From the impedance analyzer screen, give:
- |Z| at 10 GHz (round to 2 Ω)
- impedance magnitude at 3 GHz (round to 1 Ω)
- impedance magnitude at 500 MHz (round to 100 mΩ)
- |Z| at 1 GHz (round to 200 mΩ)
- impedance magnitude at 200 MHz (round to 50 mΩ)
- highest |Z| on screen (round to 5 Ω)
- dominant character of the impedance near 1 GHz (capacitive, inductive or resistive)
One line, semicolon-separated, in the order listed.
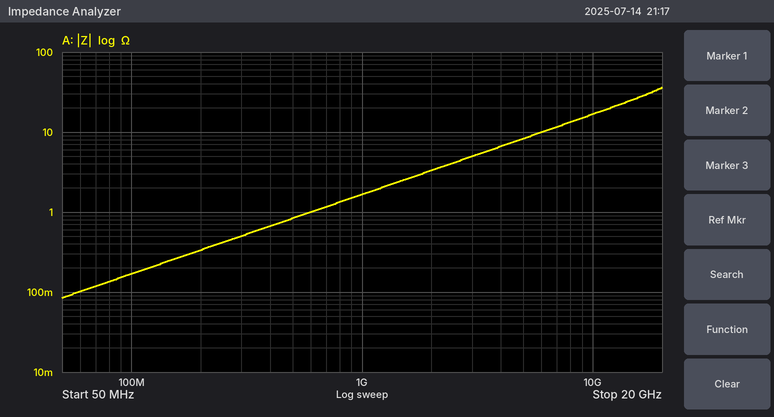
16 Ω; 5 Ω; 800 mΩ; 1.6 Ω; 350 mΩ; 35 Ω; inductive
